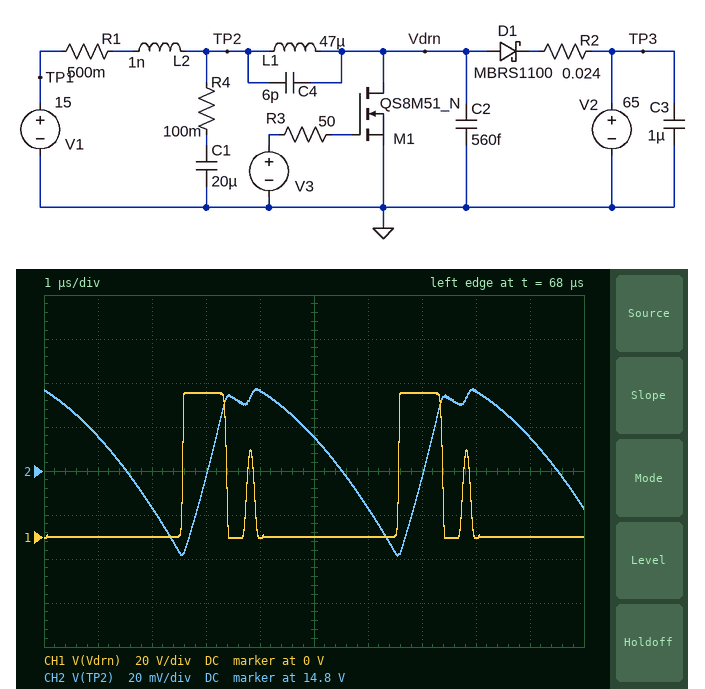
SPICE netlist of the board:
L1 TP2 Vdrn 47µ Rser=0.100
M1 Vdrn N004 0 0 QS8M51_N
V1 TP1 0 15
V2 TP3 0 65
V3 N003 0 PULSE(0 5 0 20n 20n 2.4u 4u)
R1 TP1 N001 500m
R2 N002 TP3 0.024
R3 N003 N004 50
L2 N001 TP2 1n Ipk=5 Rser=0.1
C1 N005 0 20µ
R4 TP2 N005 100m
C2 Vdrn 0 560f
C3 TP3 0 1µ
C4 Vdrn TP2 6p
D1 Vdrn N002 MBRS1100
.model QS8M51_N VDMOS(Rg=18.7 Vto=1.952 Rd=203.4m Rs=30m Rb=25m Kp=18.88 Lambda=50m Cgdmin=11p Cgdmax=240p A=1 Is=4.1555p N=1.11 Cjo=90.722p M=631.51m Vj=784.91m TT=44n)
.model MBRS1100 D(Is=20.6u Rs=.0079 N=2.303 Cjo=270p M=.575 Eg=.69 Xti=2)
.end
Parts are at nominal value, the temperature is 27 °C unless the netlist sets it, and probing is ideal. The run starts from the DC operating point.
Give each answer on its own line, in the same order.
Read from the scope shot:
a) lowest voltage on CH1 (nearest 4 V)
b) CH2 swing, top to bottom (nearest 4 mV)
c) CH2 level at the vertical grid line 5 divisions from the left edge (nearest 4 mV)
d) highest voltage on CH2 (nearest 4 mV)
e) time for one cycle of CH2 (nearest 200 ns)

0 V
76 mV
14.816 V
14.836 V
4.0 µs
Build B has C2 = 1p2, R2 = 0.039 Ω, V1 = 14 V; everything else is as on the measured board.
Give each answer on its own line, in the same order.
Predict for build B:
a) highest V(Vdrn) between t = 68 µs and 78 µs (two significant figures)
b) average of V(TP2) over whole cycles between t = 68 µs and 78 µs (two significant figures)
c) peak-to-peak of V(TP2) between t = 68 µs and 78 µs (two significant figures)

66 V
14 V
72 mV
